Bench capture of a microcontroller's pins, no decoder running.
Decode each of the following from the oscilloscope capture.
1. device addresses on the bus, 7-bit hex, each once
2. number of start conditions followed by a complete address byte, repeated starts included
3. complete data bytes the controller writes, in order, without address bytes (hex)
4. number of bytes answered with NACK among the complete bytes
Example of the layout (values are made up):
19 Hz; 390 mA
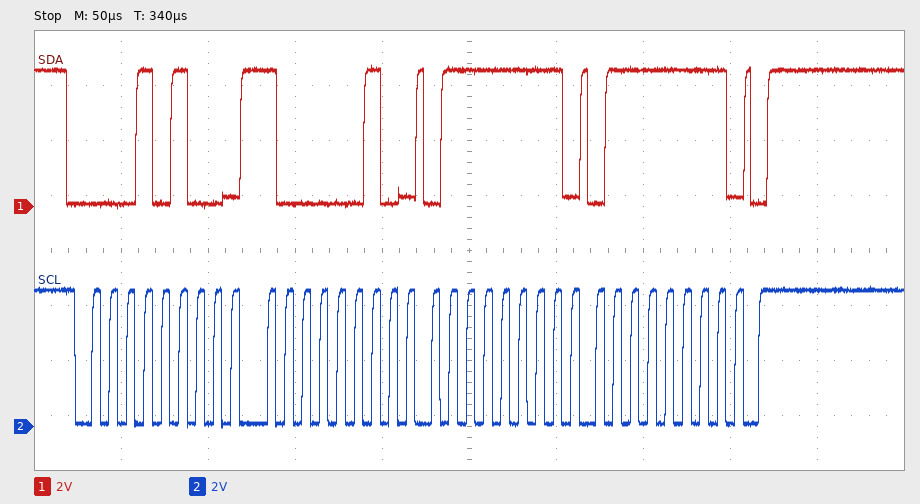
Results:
0x0A; 1; 82 7F 7F; 0
